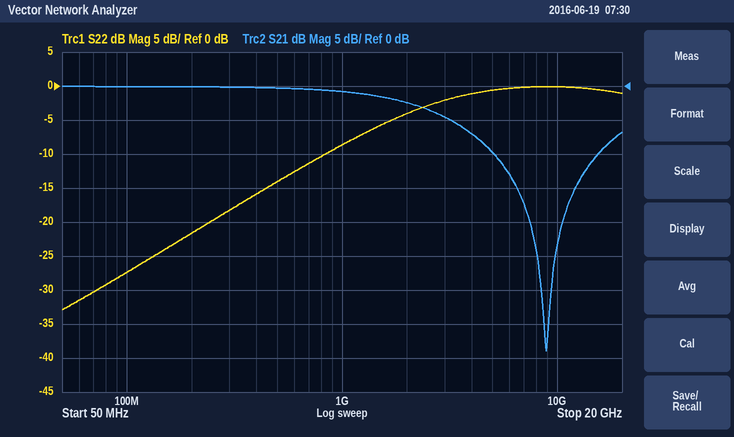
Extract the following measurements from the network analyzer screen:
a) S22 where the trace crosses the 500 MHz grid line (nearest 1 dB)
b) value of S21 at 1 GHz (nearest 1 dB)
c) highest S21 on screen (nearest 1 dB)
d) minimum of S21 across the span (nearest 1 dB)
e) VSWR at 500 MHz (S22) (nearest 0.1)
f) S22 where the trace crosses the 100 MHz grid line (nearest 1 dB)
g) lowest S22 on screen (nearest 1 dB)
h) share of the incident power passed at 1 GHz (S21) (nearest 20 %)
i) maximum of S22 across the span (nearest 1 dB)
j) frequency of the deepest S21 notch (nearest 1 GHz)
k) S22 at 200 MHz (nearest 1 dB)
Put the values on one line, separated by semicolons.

-14 dB; -1 dB; 0 dB; -39 dB; 1.5; -27 dB; -33 dB; 80 %; 0 dB; 9 GHz; -22 dB
